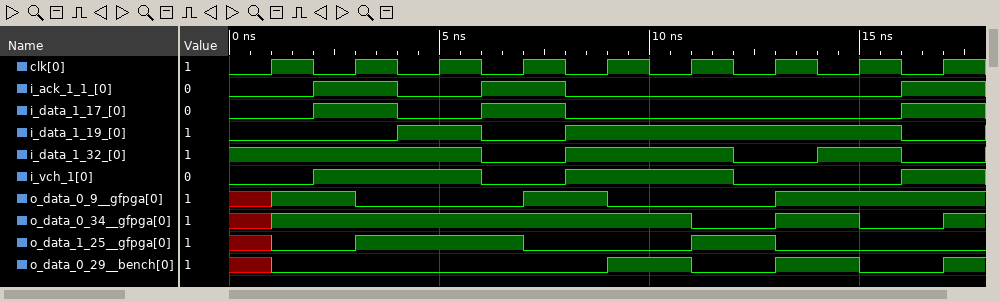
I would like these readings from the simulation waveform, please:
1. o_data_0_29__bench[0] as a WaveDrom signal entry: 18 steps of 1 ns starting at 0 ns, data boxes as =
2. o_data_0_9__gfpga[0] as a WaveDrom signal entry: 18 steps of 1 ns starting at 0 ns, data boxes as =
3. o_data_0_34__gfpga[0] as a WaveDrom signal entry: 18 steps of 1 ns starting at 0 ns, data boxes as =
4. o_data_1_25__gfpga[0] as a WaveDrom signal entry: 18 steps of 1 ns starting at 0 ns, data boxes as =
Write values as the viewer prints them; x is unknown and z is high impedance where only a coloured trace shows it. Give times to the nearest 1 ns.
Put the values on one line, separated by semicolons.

{name: 'o_data_0_29__bench[0]', wave: 'x0.......1.0.1.0.1'}; {name: 'o_data_0_9__gfpga[0]', wave: 'x1.0...1.0...1....'}; {name: 'o_data_0_34__gfpga[0]', wave: 'x1.........0.1.0.1'}; {name: 'o_data_1_25__gfpga[0]', wave: 'x0.1...0...1.0....'}
